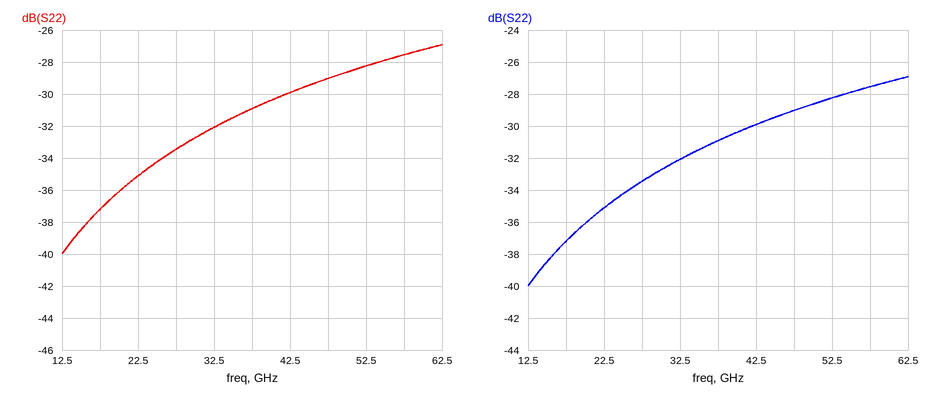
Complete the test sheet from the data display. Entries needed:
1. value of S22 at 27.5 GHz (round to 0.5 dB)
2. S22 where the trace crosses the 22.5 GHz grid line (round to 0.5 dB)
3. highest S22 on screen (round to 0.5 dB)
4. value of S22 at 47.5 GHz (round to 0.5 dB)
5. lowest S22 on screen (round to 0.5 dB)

-33.5 dB
-35.0 dB
-27.0 dB
-29.0 dB
-40.0 dB
